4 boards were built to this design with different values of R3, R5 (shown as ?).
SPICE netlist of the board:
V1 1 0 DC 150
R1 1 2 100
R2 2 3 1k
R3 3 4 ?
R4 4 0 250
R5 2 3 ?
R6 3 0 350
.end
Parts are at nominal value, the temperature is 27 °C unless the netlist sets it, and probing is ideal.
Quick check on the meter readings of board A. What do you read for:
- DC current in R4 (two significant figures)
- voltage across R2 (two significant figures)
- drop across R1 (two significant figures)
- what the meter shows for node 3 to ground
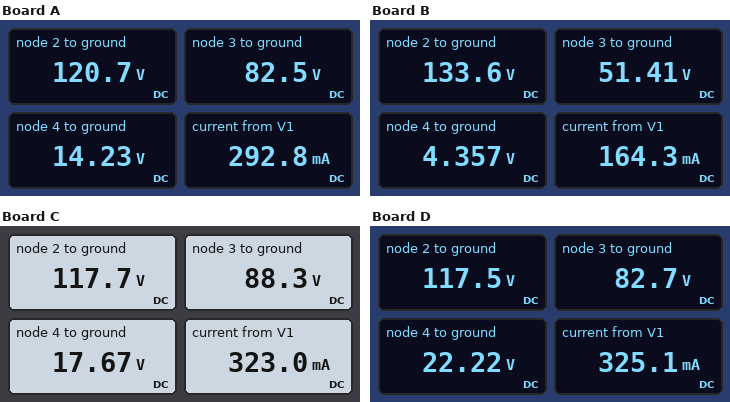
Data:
57 mA
38 V
29 V
82.5 V
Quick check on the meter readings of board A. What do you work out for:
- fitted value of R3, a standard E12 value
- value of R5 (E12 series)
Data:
1.2 kΩ
150 Ω
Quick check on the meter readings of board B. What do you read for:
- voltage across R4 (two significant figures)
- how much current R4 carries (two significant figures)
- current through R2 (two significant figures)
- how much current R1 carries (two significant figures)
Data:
4.4 V
17 mA
82 mA
160 mA
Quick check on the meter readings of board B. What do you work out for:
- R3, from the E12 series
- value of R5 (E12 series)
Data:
2.7 kΩ
1 kΩ
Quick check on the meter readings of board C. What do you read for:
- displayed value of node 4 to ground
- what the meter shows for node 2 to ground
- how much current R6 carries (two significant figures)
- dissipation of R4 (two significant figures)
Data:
17.67 V
117.7 V
250 mA
1.2 W
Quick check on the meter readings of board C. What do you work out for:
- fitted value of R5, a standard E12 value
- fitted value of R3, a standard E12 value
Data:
100 Ω
1 kΩ
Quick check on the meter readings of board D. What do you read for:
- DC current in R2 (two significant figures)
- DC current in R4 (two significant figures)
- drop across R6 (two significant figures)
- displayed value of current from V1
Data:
35 mA
89 mA
83 V
325.1 mA
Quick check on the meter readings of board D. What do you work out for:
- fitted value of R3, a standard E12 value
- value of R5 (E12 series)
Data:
680 Ω
120 Ω
